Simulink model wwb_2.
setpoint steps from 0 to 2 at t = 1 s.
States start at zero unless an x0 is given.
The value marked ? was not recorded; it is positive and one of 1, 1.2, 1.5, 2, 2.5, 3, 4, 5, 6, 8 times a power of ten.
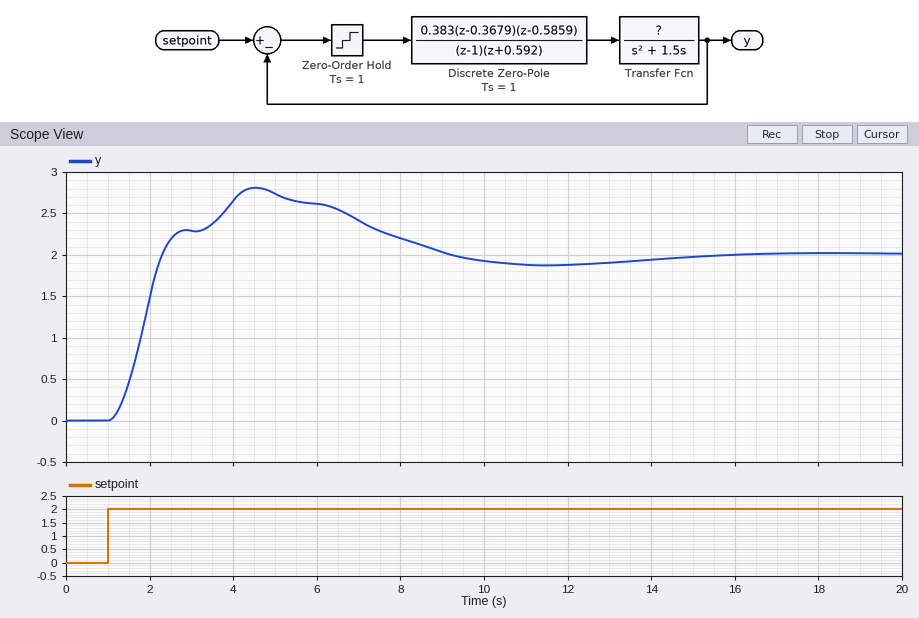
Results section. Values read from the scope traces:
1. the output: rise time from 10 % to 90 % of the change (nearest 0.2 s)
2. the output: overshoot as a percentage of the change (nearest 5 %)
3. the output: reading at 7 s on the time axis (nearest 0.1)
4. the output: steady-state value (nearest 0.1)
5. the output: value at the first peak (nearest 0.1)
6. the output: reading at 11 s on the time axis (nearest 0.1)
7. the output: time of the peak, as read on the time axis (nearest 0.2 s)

0.8 s
40 %
2.4
2.0
2.8
1.9
4.6 s
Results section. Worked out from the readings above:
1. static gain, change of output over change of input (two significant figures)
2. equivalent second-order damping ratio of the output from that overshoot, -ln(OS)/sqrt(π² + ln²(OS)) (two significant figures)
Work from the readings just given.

1.0
0.28
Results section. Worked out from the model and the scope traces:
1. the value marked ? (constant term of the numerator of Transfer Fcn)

6
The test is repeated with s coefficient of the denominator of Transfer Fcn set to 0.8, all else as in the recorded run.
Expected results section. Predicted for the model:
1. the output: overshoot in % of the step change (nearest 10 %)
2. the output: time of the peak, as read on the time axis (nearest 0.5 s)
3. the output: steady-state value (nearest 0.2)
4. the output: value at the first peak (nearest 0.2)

60 %
3.0 s
2.0
3.2
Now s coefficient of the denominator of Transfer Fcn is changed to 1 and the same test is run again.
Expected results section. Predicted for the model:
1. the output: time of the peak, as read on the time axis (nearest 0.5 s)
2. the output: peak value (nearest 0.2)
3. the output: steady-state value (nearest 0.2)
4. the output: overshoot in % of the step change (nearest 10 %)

4.0 s
3.0
2.0
50 %
